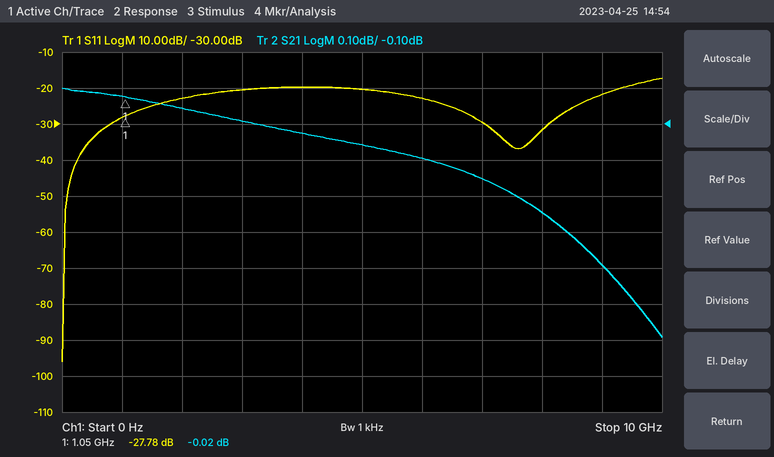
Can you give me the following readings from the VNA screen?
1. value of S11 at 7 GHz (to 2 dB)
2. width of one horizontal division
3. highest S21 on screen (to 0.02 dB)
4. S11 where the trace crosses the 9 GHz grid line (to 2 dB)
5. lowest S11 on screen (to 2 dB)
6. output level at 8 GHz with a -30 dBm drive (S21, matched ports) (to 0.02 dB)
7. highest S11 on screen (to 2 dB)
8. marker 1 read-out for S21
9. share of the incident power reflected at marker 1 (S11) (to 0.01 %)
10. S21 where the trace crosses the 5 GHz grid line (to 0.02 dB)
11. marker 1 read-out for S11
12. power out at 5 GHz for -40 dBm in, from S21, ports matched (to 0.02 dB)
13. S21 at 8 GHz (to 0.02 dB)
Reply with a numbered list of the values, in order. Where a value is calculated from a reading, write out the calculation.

1. -30 dB
2. 1 GHz
3. 0.00 dB
4. -22 dB
5. -96 dB
6. -30 dBm + (-0.34 dB) = -30.34 dBm
7. -18 dB
8. -0.02 dB
9. 10^(-27.78/10) ≈ 0.17 %
10. -0.16 dB
11. -27.78 dB
12. -40 dBm + (-0.16 dB) = -40.16 dBm
13. -0.34 dB
